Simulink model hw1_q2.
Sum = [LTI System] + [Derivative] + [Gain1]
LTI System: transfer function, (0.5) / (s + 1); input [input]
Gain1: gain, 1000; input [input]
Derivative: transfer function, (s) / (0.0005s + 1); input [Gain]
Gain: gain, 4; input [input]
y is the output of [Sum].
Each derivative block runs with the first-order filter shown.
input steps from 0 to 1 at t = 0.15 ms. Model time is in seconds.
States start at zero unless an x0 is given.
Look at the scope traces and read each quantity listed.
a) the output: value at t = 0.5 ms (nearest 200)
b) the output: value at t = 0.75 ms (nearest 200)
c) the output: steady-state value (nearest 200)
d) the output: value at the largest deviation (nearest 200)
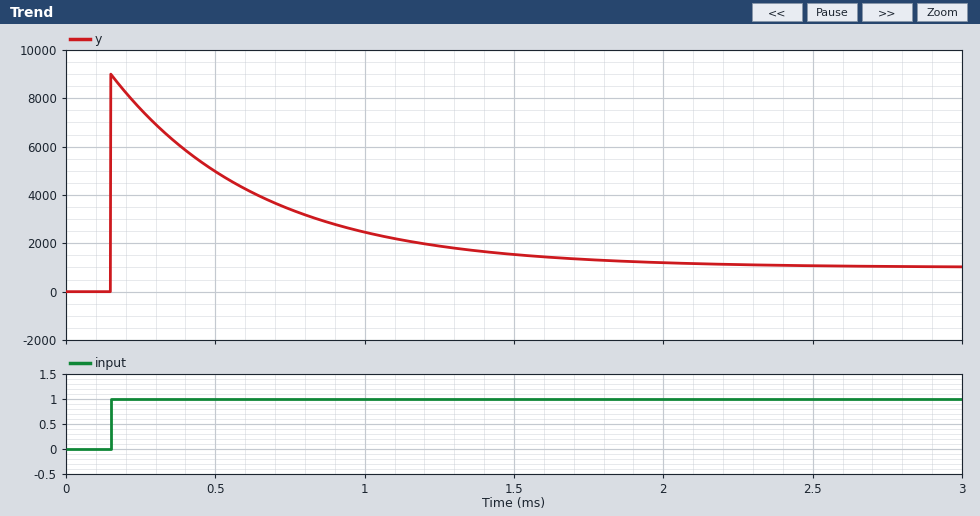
5000
3400
1000
9000
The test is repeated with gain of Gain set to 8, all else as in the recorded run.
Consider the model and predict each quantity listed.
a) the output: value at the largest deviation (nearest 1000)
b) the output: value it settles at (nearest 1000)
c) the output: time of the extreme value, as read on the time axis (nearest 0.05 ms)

17000
1000
0.15 ms
